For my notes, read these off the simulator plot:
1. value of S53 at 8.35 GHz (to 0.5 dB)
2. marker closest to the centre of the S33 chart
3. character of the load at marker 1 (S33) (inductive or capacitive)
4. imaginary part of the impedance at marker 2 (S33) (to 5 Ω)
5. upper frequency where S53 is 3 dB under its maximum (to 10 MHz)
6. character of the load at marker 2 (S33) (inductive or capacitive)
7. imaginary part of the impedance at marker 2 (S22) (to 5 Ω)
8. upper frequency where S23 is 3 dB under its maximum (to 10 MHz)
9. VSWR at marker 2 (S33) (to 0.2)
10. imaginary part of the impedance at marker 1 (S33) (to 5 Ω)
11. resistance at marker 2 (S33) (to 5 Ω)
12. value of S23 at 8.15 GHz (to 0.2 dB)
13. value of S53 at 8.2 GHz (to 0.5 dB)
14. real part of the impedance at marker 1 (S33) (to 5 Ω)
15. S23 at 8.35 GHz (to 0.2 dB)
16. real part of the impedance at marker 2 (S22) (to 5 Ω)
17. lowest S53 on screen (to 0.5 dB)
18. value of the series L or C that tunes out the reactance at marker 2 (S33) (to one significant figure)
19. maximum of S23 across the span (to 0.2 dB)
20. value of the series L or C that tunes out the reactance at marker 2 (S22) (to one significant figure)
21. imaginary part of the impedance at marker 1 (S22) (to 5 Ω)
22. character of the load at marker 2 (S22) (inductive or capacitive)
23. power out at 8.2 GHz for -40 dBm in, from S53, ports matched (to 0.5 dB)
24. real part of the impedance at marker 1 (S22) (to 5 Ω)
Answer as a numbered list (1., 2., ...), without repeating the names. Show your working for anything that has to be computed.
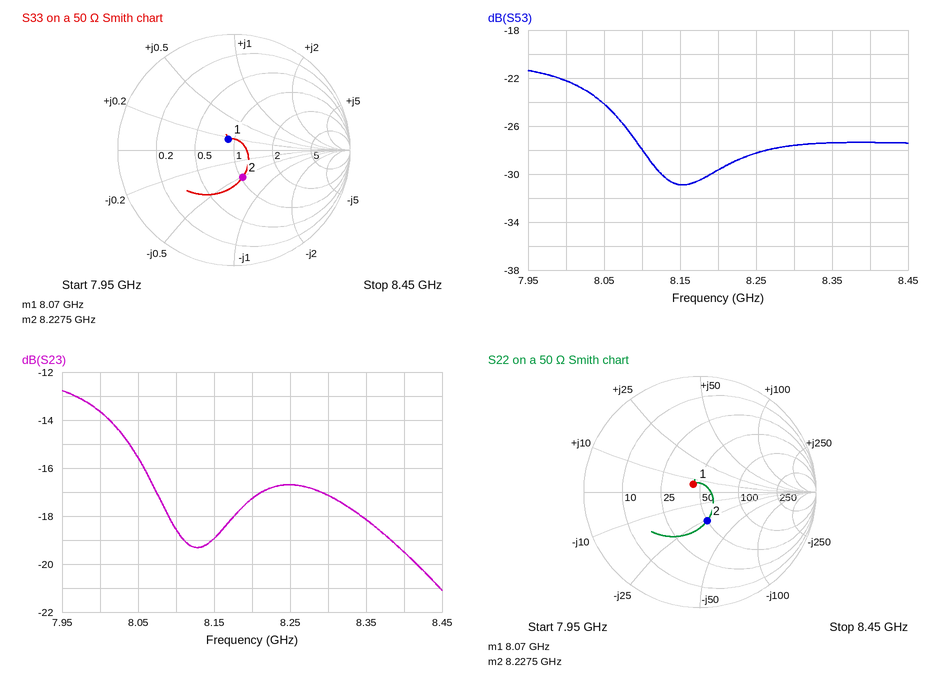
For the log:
1. -27.5 dB
2. marker 1
3. inductive
4. -25 Ω
5. 8.05 GHz
6. capacitive
7. -25 Ω
8. 8.05 GHz
9. 1.6
10. +10 Ω
11. 50 Ω
12. -19.0 dB
13. -29.5 dB
14. 45 Ω
15. -18.2 dB
16. 50 Ω
17. -31.0 dB
18. L = 25 Ω/(2π × 8.2275 GHz) ≈ 484 pH, so 500 pH to one significant figure
19. -12.8 dB
20. L = 25 Ω/(2π × 8.2275 GHz) ≈ 484 pH, so 500 pH to one significant figure
21. +5 Ω
22. capacitive
23. -40 dBm + (-29.5 dB) = -69.5 dBm
24. 45 Ω
